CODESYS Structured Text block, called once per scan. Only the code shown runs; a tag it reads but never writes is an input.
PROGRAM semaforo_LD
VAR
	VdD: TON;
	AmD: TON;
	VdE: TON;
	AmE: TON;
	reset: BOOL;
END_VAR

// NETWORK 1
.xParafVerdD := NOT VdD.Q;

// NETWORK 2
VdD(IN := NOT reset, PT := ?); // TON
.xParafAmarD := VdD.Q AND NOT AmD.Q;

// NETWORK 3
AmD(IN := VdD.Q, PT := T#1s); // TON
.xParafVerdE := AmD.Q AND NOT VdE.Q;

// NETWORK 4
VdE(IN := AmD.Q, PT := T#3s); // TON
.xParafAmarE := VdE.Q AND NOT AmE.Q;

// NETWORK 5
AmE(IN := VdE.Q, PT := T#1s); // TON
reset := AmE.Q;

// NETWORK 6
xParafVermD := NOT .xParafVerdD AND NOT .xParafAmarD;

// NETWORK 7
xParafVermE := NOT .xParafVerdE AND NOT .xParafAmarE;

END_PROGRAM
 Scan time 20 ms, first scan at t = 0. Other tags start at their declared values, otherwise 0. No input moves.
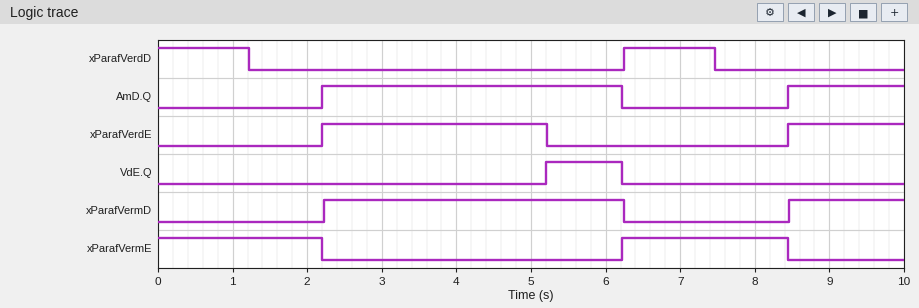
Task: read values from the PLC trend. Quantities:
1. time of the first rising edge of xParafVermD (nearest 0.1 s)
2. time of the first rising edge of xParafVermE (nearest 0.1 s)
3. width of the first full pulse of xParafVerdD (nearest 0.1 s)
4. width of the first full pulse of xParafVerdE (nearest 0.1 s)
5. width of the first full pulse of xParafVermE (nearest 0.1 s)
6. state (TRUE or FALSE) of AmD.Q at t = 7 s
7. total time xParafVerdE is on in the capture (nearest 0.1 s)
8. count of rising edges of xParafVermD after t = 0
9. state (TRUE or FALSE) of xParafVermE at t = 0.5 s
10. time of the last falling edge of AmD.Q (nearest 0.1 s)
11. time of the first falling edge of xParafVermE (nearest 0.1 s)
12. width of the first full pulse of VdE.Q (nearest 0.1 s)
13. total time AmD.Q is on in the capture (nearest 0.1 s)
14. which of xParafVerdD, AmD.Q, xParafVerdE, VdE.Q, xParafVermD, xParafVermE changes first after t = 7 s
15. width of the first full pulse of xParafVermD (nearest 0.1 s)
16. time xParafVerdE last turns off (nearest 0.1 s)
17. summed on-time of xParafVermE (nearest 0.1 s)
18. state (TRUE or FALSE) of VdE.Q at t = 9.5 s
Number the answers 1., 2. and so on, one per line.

1. 2.2 s
2. 6.2 s
3. 1.2 s
4. 3.0 s
5. 2.2 s
6. FALSE
7. 4.6 s
8. 2
9. TRUE
10. 6.2 s
11. 2.2 s
12. 1.0 s
13. 5.6 s
14. xParafVerdD
15. 4.0 s
16. 5.2 s
17. 4.4 s
18. FALSE
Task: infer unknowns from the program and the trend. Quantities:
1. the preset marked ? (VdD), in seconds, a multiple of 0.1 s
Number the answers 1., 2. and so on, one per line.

1. 1.2 s
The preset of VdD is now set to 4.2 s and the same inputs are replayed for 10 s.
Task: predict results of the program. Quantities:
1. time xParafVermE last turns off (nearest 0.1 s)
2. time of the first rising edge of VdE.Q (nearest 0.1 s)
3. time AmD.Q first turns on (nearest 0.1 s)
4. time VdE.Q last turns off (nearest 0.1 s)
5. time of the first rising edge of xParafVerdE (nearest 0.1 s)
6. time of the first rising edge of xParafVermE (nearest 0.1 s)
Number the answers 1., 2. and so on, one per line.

1. 5.2 s
2. 8.2 s
3. 5.2 s
4. 9.2 s
5. 5.2 s
6. 9.2 s
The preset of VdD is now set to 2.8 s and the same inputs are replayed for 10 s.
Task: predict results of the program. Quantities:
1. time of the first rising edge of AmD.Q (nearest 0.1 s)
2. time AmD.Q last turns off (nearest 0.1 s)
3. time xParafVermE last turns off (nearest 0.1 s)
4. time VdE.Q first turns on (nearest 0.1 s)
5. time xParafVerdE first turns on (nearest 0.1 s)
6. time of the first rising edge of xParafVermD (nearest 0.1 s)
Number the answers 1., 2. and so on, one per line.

1. 3.8 s
2. 7.8 s
3. 3.8 s
4. 6.8 s
5. 3.8 s
6. 3.8 s
